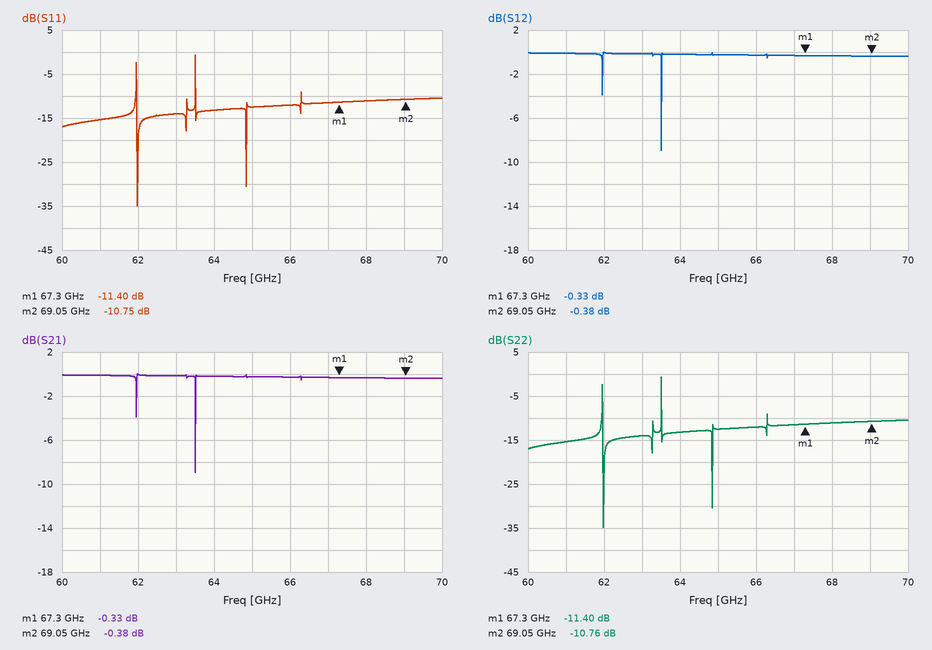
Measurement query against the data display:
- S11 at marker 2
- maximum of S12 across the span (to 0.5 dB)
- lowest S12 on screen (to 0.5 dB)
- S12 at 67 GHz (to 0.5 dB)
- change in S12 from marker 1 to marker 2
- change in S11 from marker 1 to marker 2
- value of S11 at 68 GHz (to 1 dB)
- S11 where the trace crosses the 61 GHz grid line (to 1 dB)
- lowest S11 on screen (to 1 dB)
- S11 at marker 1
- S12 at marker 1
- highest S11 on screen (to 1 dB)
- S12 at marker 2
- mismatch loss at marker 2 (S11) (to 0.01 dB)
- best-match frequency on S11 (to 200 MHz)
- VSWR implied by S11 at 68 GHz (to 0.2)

-10.75 dB
0.0 dB
-9.0 dB
-0.5 dB
-0.05 dB
0.65 dB
-11 dB
-15 dB
-35 dB
-11.40 dB
-0.33 dB
-1 dB
-0.38 dB
0.38 dB
62.0 GHz
1.8
